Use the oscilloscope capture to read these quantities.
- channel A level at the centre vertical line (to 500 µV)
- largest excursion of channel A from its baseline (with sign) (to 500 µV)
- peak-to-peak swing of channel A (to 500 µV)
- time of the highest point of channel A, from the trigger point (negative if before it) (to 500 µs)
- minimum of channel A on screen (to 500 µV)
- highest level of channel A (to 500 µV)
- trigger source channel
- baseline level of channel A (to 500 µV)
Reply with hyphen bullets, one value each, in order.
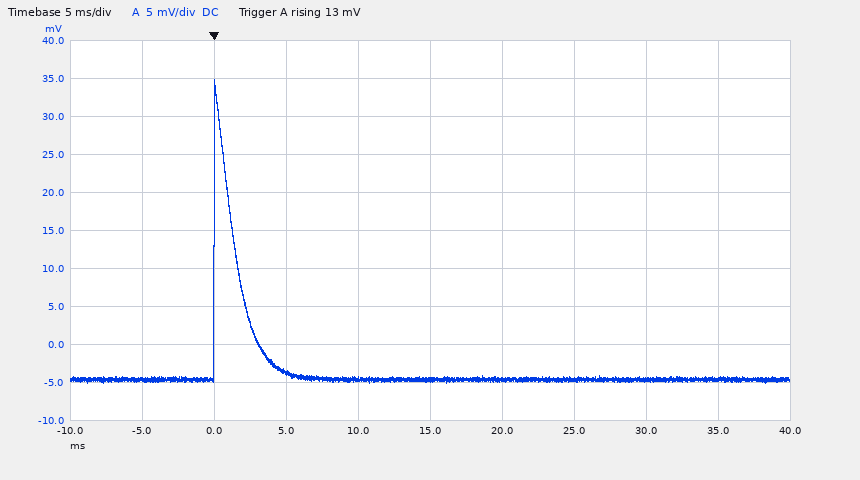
- -4.5 mV
- +39.5 mV
- 40.0 mV
- 0.0 ms
- -5.0 mV
- 35.0 mV
- channel A
- -4.5 mV
